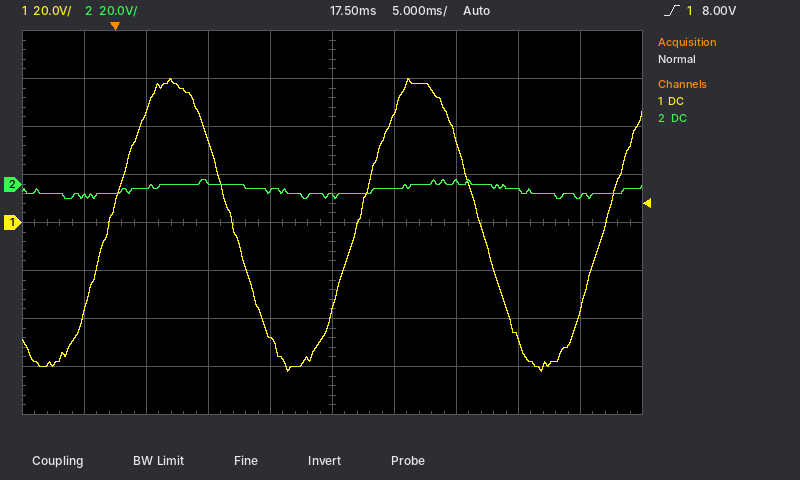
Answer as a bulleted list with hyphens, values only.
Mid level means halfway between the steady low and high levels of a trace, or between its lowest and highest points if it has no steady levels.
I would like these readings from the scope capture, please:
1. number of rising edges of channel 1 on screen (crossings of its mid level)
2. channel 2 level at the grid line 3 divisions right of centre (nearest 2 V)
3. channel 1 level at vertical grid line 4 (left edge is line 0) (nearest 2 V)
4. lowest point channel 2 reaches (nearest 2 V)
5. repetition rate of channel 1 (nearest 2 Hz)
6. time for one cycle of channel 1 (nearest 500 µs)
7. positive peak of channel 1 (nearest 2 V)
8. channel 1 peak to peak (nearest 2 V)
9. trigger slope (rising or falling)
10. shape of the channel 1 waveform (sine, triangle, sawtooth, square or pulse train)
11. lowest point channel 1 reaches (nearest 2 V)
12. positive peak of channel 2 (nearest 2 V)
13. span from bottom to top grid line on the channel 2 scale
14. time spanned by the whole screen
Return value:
- 3
- -2 V
- -48 V
- -6 V
- 50 Hz
- 20.0 ms
- 60 V
- 122 V
- rising
- sine
- -62 V
- 2 V
- 160 V
- 50 ms
